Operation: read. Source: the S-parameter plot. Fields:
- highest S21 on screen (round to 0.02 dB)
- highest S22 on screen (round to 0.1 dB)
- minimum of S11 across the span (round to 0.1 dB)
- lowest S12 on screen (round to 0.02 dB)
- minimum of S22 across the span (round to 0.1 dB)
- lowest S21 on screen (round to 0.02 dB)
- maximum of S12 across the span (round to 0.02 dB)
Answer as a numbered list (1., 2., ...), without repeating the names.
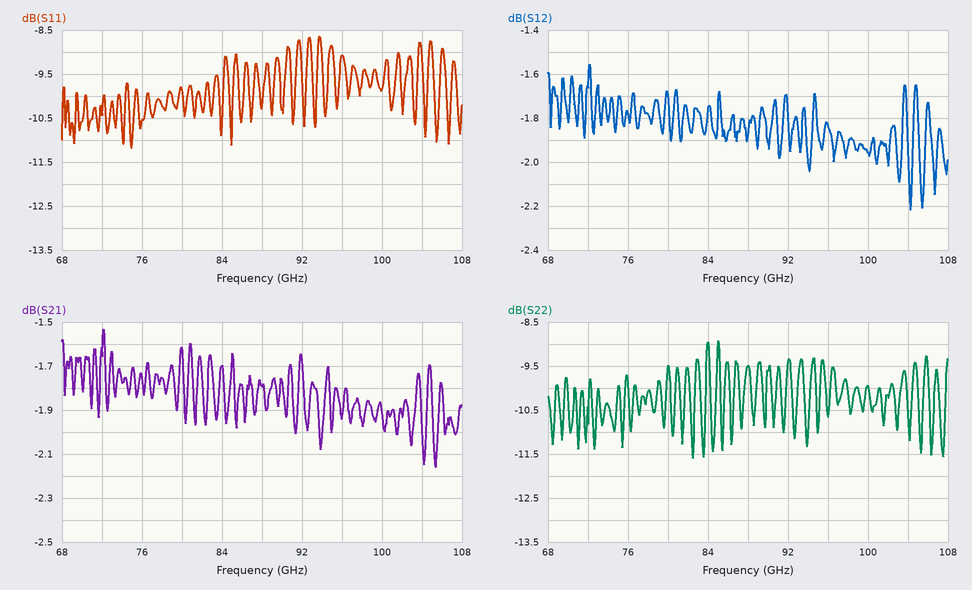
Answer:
1. -1.54 dB
2. -8.9 dB
3. -11.2 dB
4. -2.22 dB
5. -11.6 dB
6. -2.16 dB
7. -1.56 dB
